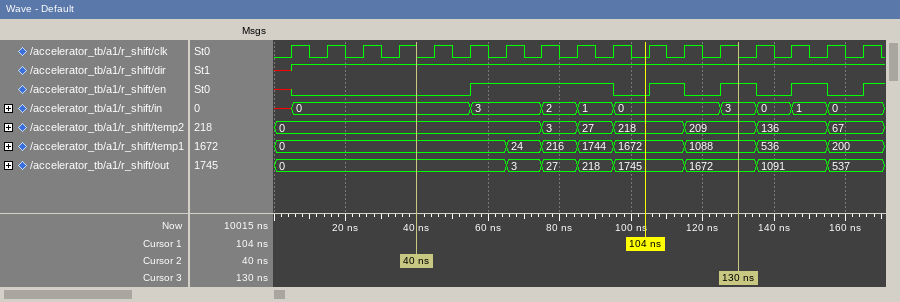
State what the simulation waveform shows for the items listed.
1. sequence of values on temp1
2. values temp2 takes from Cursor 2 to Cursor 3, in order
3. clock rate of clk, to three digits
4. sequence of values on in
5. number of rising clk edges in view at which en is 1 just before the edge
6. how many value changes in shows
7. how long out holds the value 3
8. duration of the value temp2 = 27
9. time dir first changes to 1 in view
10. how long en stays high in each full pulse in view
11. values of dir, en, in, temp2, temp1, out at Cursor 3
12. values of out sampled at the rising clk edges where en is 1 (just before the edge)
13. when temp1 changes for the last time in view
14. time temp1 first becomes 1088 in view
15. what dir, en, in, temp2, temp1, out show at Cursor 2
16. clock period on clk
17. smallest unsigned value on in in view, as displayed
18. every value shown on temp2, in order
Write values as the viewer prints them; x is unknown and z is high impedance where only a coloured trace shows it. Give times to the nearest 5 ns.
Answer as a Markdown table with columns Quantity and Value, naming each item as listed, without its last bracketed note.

| Quantity | Value |
|---|---|
| sequence of values on temp1 | 0, 24, 216, 1744, 1672, 1088, 536, 200 |
| values temp2 takes from Cursor 2 to Cursor 3, in order | 0, 3, 27, 218, 209 |
| clock rate of clk, to three digits | 100 MHz |
| sequence of values on in | x, 0, 3, 2, 1, 0, 3, 0, 1, 0 |
| number of rising clk edges in view at which en is 1 just before the edge | 7 |
| how many value changes in shows | 9 |
| how long out holds the value 3 | 10 ns |
| duration of the value temp2 = 27 | 10 ns |
| time dir first changes to 1 in view | 5 ns |
| how long en stays high in each full pulse in view | 40 ns, 10 ns, 10 ns, 10 ns |
| values of dir, en, in, temp2, temp1, out at Cursor 3 | dir=1, en=1, in=3, temp2=209, temp1=1088, out=1672 |
| values of out sampled at the rising clk edges where en is 1 | 0, 3, 27, 218, 1745, 1672, 1091 |
| when temp1 changes for the last time in view | 155 ns |
| time temp1 first becomes 1088 in view | 115 ns |
| what dir, en, in, temp2, temp1, out show at Cursor 2 | dir=1, en=0, in=0, temp2=0, temp1=0, out=0 |
| clock period on clk | 10 ns |
| smallest unsigned value on in in view, as displayed | 0 |
| every value shown on temp2, in order | 0, 3, 27, 218, 209, 136, 67 |
